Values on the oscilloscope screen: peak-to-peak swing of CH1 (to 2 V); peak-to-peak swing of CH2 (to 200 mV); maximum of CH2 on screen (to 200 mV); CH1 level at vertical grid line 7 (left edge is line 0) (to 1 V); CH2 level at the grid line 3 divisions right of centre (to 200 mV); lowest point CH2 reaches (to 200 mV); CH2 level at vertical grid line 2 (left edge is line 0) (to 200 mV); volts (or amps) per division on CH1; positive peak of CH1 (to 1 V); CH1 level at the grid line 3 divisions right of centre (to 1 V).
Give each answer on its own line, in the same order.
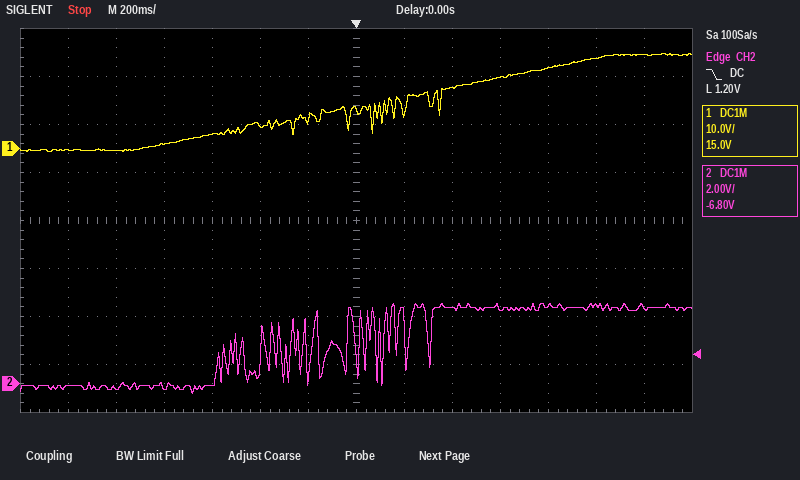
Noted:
20 V
3.8 V
3.4 V
8 V
3.2 V
-400 mV
-200 mV
10 V
20 V
15 V
